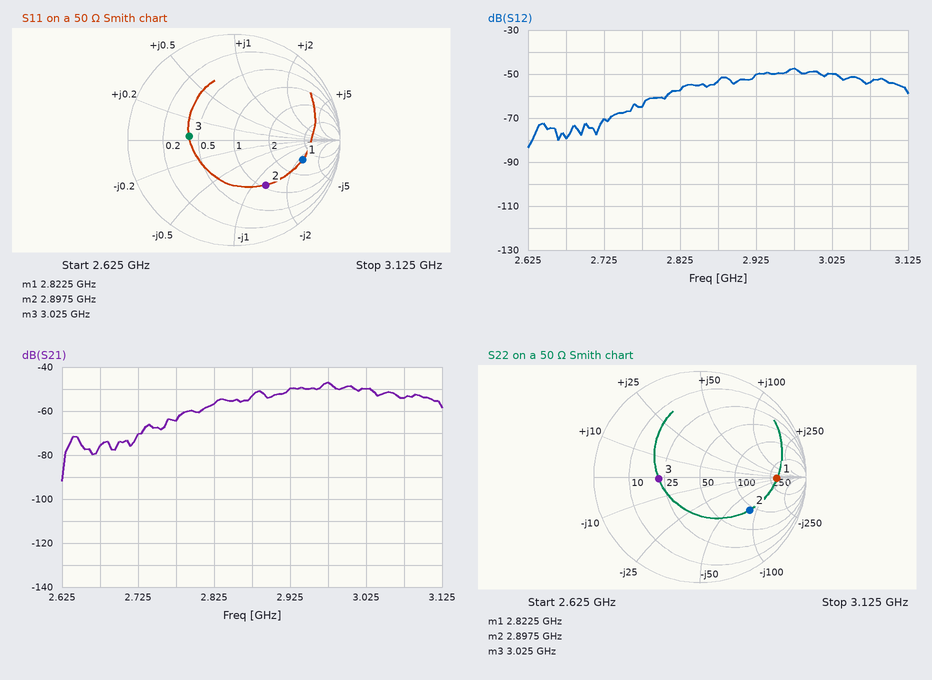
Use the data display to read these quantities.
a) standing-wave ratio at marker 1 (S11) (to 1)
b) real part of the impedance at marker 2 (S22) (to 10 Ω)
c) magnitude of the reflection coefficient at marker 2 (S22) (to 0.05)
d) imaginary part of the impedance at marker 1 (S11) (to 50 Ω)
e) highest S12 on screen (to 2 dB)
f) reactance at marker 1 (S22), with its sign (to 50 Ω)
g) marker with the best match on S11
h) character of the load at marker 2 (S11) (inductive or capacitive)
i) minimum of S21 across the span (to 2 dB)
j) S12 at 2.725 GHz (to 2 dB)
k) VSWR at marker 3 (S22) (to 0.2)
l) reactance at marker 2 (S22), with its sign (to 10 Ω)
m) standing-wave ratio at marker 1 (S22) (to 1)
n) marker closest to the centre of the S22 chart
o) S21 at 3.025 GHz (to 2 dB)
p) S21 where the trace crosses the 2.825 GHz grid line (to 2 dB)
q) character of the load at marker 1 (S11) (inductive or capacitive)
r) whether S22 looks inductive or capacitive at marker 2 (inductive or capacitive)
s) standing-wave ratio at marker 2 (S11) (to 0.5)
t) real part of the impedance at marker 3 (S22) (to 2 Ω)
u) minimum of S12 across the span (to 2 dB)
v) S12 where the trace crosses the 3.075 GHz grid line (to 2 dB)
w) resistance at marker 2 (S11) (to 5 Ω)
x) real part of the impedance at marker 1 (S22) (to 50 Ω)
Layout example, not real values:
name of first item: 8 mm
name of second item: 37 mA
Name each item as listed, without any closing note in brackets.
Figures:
standing-wave ratio at marker 1 (S11): 5
real part of the impedance at marker 2 (S22): 90 Ω
magnitude of the reflection coefficient at marker 2 (S22): 0.55
imaginary part of the impedance at marker 1 (S11): -100 Ω
highest S12 on screen: -48 dB
reactance at marker 1 (S22), with its sign: 0 Ω
marker with the best match on S11: marker 3
character of the load at marker 2 (S11): capacitive
minimum of S21 across the span: -92 dB
S12 at 2.725 GHz: -70 dB
VSWR at marker 3 (S22): 2.2
reactance at marker 2 (S22), with its sign: -80 Ω
standing-wave ratio at marker 1 (S22): 6
marker closest to the centre of the S22 chart: marker 3
S21 at 3.025 GHz: -50 dB
S21 where the trace crosses the 2.825 GHz grid line: -56 dB
character of the load at marker 1 (S11): capacitive
whether S22 looks inductive or capacitive at marker 2: capacitive
standing-wave ratio at marker 2 (S11): 3.0
real part of the impedance at marker 3 (S22): 22 Ω
minimum of S12 across the span: -84 dB
S12 where the trace crosses the 3.075 GHz grid line: -54 dB
resistance at marker 2 (S11): 55 Ω
real part of the impedance at marker 1 (S22): 300 Ω
